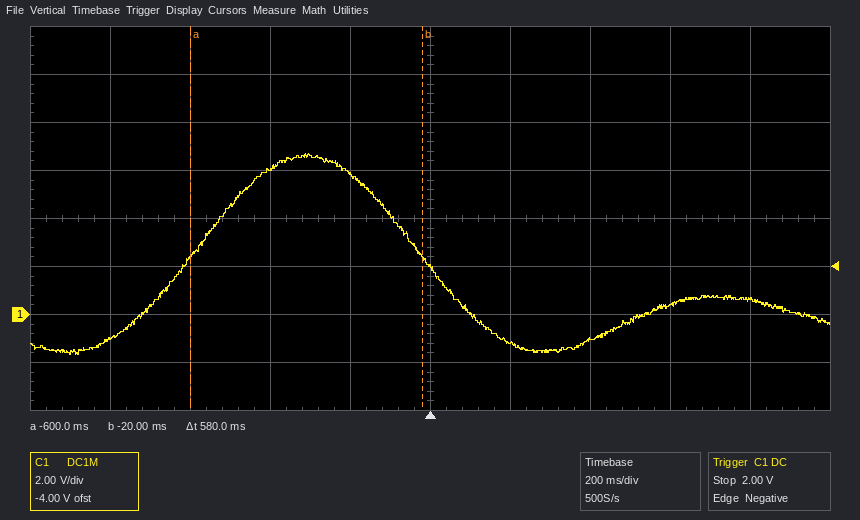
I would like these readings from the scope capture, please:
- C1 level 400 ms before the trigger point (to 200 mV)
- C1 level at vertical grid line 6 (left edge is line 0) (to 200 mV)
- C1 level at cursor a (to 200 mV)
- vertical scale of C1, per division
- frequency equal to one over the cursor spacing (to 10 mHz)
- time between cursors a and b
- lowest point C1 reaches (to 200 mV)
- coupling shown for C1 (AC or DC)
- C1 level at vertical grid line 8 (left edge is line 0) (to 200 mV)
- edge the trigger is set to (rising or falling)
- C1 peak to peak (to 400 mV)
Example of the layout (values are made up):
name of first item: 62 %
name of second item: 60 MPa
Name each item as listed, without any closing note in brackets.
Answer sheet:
C1 level 400 ms before the trigger point: 6.0 V
C1 level at vertical grid line 6 (left edge is line 0): -1.2 V
C1 level at cursor a: 2.4 V
vertical scale of C1, per division: 2 V
frequency equal to one over the cursor spacing: 1.72 Hz
time between cursors a and b: 580 ms
lowest point C1 reaches: -1.6 V
coupling shown for C1: DC
C1 level at vertical grid line 8 (left edge is line 0): 400 mV
edge the trigger is set to: falling
C1 peak to peak: 8.4 V
